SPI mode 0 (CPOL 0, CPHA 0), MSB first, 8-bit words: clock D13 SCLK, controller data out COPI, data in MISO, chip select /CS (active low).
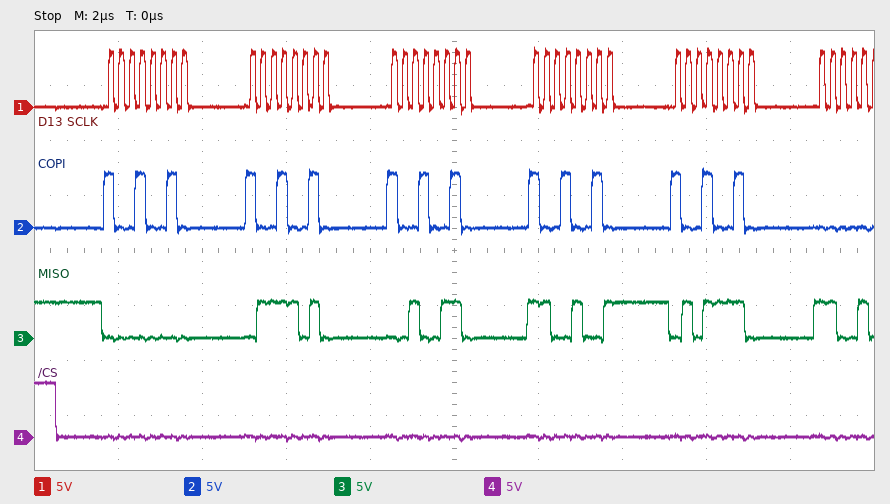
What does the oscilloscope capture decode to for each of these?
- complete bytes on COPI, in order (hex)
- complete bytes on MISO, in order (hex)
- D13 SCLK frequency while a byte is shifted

92 92 92 92 92
00 7A 26 C9 5E
4 MHz
